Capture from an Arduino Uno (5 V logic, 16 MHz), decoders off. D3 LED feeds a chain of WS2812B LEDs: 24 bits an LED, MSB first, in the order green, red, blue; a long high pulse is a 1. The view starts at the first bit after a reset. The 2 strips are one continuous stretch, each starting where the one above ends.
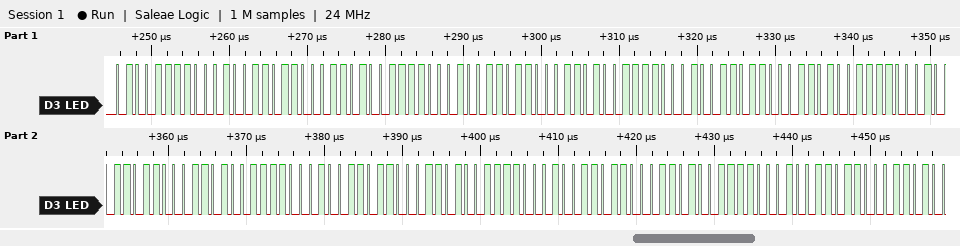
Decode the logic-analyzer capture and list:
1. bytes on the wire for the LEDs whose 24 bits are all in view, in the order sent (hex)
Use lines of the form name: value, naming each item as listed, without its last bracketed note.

bytes on the wire for the LEDs whose 24 bits are all in view, in the order sent: 4F 13 63 4F 13 63 4F 13 63 4F 13 63 4F 13 63 4F 13 63 4F 13 63
